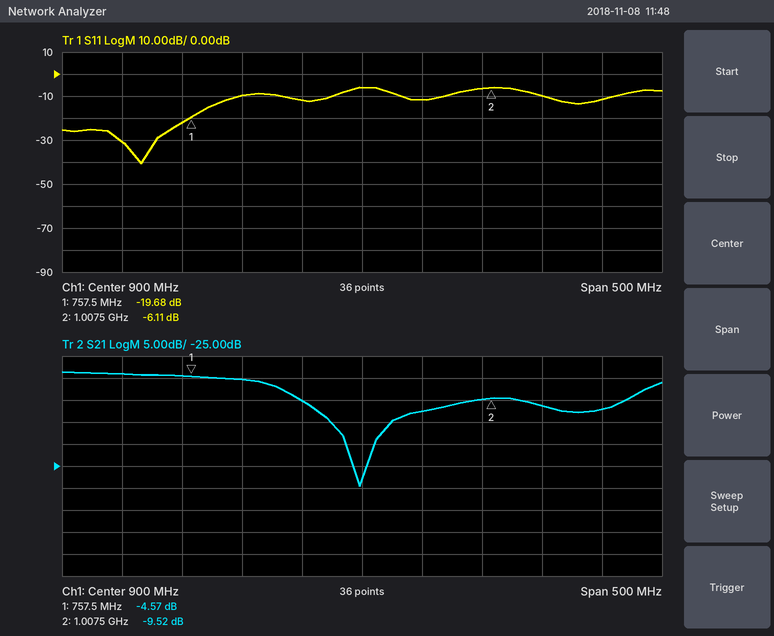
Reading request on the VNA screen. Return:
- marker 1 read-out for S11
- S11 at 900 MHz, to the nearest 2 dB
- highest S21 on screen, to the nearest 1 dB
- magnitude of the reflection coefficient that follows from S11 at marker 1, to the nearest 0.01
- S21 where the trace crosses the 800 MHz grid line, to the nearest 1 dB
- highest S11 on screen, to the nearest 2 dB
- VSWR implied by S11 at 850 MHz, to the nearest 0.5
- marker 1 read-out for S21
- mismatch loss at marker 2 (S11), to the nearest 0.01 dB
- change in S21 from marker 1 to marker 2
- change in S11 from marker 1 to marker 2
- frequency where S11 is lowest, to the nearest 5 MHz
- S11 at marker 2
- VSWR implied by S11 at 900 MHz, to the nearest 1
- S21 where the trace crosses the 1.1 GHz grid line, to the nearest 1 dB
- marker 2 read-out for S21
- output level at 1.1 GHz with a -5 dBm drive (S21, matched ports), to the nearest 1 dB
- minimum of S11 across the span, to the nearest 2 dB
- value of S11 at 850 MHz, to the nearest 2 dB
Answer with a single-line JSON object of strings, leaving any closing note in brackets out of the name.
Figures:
{"marker 1 read-out for S11": "-19.68 dB", "S11 at 900 MHz, to the nearest 2 dB": "-6 dB", "highest S21 on screen, to the nearest 1 dB": "-4 dB", "magnitude of the reflection coefficient that follows from S11 at marker 1, to the nearest 0.01": "0.10", "S21 where the trace crosses the 800 MHz grid line, to the nearest 1 dB": "-5 dB", "highest S11 on screen, to the nearest 2 dB": "-6 dB", "VSWR implied by S11 at 850 MHz, to the nearest 0.5": "1.5", "marker 1 read-out for S21": "-4.57 dB", "mismatch loss at marker 2 (S11), to the nearest 0.01 dB": "1.22 dB", "change in S21 from marker 1 to marker 2": "-4.95 dB", "change in S11 from marker 1 to marker 2": "13.57 dB", "frequency where S11 is lowest, to the nearest 5 MHz": "715 MHz", "S11 at marker 2": "-6.11 dB", "VSWR implied by S11 at 900 MHz, to the nearest 1": "3", "S21 where the trace crosses the 1.1 GHz grid line, to the nearest 1 dB": "-12 dB", "marker 2 read-out for S21": "-9.52 dB", "output level at 1.1 GHz with a -5 dBm drive (S21, matched ports), to the nearest 1 dB": "-17 dBm", "minimum of S11 across the span, to the nearest 2 dB": "-40 dB", "value of S11 at 850 MHz, to the nearest 2 dB": "-12 dB"}
